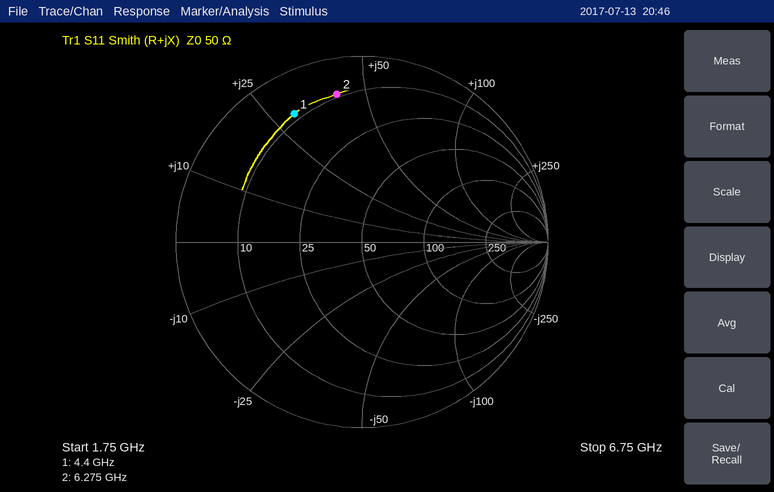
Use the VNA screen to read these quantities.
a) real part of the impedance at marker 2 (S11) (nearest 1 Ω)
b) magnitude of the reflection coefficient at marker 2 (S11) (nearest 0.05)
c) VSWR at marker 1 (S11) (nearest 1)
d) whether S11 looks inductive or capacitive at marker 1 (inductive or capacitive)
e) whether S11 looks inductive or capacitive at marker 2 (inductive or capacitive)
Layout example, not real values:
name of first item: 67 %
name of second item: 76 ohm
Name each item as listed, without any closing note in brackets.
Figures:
real part of the impedance at marker 2 (S11): 9 Ω
magnitude of the reflection coefficient at marker 2 (S11): 0.80
VSWR at marker 1 (S11): 8
whether S11 looks inductive or capacitive at marker 1: inductive
whether S11 looks inductive or capacitive at marker 2: inductive
